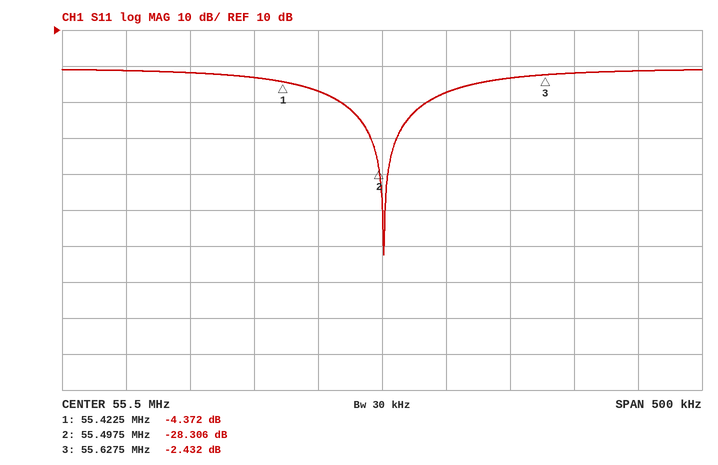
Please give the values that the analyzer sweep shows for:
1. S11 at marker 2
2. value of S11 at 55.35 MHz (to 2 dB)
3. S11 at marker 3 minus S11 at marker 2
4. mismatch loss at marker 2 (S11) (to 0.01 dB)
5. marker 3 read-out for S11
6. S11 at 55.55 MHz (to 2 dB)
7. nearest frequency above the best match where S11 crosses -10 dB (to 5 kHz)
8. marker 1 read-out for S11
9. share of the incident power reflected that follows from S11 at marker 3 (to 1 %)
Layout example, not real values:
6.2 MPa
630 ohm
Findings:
-28.306 dB
-2 dB
25.874 dB
0.01 dB
-2.432 dB
-8 dB
55.535 MHz
-4.372 dB
57 %
